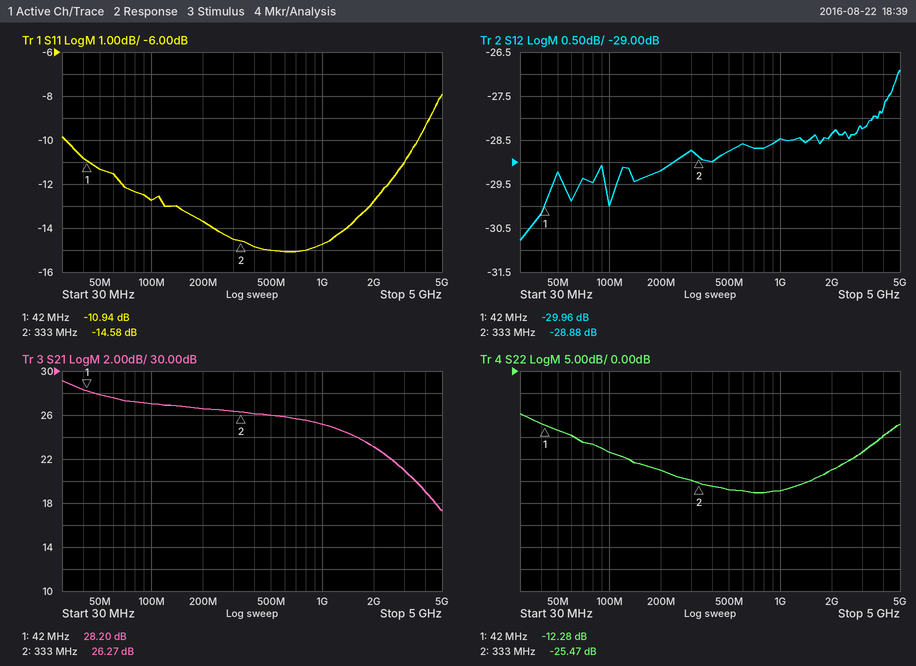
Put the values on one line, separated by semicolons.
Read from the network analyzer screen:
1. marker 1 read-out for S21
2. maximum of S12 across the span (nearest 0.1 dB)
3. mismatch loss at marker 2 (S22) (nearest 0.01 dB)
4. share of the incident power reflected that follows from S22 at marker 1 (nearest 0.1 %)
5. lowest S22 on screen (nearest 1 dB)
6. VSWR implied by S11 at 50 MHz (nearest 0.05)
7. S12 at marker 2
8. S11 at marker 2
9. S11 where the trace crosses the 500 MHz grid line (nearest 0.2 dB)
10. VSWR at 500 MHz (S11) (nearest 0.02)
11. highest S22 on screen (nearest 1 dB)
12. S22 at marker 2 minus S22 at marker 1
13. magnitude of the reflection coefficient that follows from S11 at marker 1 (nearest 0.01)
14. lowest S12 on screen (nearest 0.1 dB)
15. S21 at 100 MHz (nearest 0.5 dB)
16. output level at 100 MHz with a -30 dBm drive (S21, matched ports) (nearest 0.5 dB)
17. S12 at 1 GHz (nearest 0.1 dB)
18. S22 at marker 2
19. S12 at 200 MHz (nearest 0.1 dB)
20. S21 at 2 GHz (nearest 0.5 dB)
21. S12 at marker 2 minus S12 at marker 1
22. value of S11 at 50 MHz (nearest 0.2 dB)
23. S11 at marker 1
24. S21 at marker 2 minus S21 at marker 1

28.20 dB; -26.9 dB; 0.01 dB; 5.9 %; -28 dB; 1.75; -28.88 dB; -14.58 dB; -15.0 dB; 1.44; -10 dB; -13.19 dB; 0.28; -30.8 dB; 27.0 dB; -3.0 dBm; -28.5 dB; -25.47 dB; -29.2 dB; 23.0 dB; 1.08 dB; -11.4 dB; -10.94 dB; -1.93 dB
